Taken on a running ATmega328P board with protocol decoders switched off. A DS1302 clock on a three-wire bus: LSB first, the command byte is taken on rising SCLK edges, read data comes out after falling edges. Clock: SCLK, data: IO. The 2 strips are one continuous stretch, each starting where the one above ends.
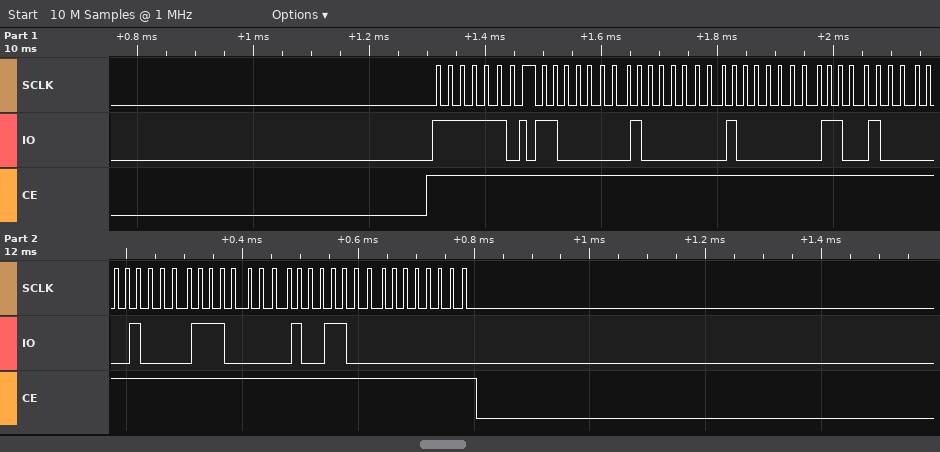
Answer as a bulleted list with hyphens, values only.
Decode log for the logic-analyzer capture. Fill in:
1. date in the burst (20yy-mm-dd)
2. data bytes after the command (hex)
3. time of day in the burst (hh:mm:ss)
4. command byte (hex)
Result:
- 2019-08-13
- 03 01 01 13 08 07 19 00
- 01:01:03
- 0xBF
